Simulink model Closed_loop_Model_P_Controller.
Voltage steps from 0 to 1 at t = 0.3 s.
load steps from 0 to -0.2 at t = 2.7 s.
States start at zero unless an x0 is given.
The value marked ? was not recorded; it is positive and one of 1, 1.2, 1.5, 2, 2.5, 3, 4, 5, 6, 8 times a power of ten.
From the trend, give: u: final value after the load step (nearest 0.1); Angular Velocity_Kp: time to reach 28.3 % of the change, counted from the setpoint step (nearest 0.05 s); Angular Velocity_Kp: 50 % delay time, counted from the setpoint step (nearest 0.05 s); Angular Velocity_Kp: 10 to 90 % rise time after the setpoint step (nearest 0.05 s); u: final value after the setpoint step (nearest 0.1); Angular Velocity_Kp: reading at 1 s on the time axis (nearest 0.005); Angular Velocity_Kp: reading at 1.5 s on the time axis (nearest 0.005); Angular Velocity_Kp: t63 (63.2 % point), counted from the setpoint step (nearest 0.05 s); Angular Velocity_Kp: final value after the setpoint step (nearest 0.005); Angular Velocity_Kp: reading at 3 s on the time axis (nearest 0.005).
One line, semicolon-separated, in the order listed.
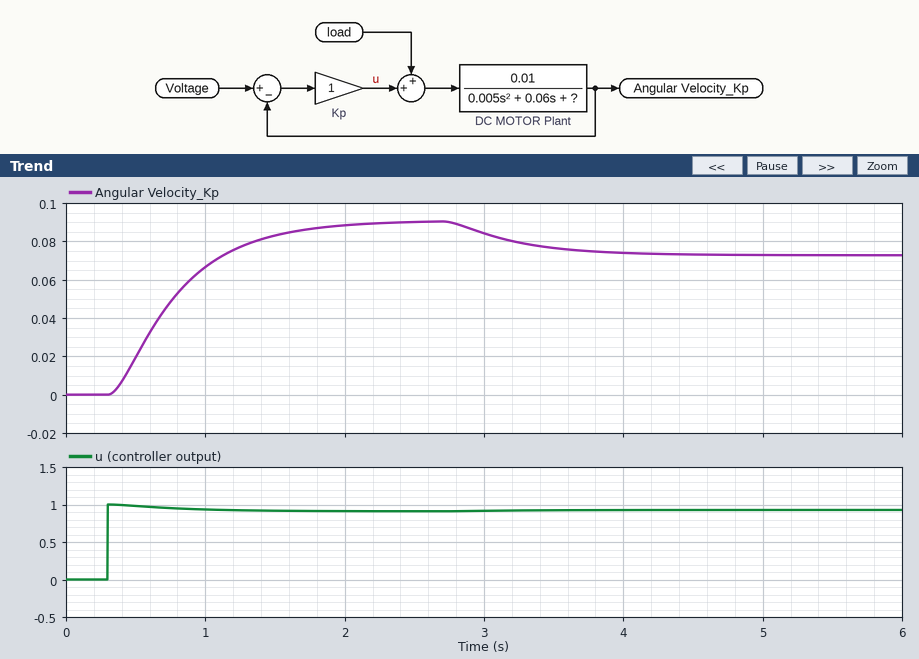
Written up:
0.9; 0.25 s; 0.40 s; 1.00 s; 0.9; 0.065; 0.085; 0.55 s; 0.090; 0.085
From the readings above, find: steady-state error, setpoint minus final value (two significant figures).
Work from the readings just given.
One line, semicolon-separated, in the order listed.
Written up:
0.91
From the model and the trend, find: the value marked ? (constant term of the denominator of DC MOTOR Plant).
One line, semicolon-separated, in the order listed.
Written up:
0.1
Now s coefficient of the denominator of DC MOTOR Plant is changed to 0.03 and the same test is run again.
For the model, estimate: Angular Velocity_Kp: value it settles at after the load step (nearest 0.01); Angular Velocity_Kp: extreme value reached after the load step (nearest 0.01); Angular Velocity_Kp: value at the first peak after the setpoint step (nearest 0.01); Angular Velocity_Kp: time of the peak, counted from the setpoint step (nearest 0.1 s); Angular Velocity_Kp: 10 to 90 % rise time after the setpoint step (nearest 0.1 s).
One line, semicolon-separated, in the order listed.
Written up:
0.07; 0.07; 0.10; 0.9 s; 0.4 s
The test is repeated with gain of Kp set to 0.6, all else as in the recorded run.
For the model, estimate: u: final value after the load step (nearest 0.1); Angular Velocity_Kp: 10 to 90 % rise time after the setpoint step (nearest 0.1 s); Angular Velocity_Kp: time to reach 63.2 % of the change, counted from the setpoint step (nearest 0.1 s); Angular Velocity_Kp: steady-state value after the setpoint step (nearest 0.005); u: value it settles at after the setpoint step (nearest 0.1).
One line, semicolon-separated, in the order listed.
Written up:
0.6; 1.1 s; 0.6 s; 0.055; 0.6
